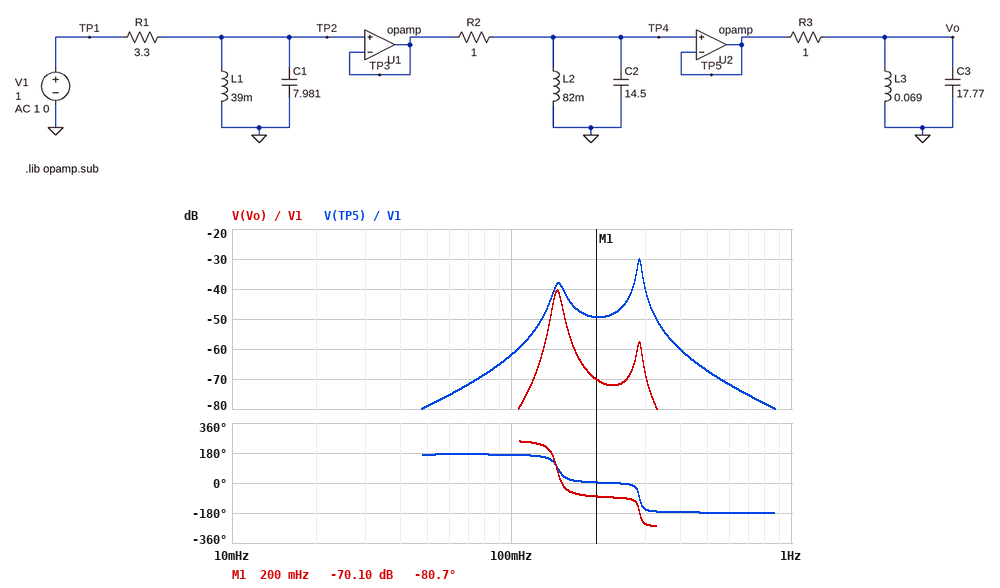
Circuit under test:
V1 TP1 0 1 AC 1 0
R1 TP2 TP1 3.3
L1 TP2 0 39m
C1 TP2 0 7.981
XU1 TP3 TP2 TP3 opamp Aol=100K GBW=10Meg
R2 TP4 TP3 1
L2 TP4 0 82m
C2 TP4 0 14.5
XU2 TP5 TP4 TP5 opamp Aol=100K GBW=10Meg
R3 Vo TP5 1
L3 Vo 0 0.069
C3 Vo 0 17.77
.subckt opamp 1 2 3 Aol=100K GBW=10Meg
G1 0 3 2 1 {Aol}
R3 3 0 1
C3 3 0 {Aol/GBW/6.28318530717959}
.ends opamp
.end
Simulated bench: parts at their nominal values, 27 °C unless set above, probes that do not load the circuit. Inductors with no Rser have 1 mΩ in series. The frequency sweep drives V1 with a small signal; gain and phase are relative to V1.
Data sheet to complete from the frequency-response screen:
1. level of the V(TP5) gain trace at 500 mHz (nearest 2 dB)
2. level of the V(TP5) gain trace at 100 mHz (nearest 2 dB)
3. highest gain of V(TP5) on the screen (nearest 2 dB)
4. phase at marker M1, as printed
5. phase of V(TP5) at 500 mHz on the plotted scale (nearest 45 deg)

-68 dB
-62 dB
-30 dB
-80.7 deg
-180 deg
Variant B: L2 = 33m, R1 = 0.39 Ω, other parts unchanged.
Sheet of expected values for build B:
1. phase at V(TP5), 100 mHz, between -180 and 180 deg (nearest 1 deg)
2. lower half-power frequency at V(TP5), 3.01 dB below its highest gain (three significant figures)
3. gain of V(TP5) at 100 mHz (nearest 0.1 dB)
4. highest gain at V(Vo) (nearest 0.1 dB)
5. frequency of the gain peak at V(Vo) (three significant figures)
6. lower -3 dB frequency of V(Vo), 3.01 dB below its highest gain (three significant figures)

168 deg
224 mHz
-54.8 dB
-35.6 dB
231 mHz
223 mHz
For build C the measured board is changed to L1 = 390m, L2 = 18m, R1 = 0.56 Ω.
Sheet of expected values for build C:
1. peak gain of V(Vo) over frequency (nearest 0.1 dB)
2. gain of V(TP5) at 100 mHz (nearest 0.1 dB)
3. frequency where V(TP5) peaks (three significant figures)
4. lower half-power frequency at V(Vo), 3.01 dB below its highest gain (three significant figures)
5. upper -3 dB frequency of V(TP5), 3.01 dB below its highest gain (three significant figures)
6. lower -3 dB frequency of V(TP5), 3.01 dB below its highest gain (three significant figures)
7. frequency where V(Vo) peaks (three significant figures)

-44.1 dB
-39.1 dB
311 mHz
138 mHz
321 mHz
301 mHz
144 mHz
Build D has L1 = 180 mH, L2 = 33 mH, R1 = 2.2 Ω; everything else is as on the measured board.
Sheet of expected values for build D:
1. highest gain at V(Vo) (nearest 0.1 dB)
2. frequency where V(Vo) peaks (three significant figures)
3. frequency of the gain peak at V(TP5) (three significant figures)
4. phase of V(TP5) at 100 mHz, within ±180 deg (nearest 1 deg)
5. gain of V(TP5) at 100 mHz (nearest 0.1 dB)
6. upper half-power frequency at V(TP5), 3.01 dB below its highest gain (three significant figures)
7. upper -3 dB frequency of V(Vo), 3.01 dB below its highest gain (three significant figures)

-35.9 dB
141 mHz
230 mHz
167 deg
-50.4 dB
237 mHz
147 mHz
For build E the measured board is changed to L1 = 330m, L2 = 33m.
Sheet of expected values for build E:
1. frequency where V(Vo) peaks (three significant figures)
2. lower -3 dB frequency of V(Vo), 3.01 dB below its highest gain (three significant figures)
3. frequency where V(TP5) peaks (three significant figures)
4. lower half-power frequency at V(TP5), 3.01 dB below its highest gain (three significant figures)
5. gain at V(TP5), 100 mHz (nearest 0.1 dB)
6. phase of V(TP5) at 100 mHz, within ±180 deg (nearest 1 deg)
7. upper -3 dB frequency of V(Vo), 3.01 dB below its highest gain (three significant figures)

144 mHz
138 mHz
98.2 mHz
95.2 mHz
-33.8 dB
55 deg
149 mHz
